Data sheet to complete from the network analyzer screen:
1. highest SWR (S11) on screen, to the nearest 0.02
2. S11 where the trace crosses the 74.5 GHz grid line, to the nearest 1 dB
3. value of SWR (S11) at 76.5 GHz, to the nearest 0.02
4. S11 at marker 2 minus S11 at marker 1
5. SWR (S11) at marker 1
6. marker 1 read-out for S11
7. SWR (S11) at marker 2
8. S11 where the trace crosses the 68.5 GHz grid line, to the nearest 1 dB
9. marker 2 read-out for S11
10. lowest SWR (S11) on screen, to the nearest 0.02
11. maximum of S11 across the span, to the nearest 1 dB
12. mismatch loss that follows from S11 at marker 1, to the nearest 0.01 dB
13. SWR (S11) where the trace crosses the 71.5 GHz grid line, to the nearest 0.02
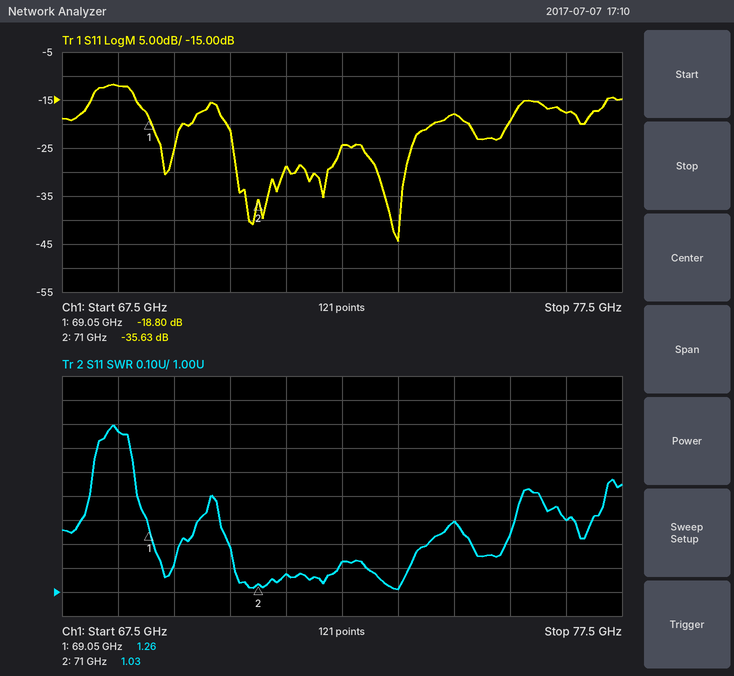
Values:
1.70
-18 dB
1.30
-16.83 dB
1.26
-18.80 dB
1.03
-12 dB
-35.63 dB
1.02
-12 dB
0.06 dB
1.08
